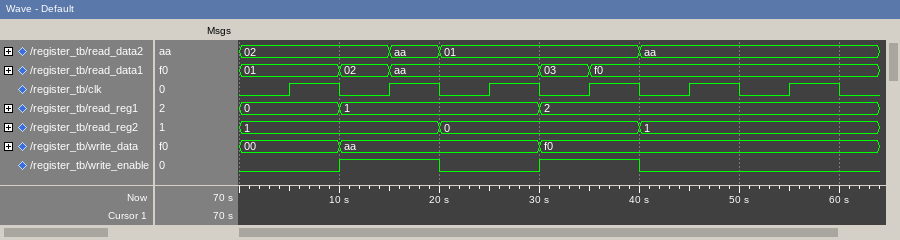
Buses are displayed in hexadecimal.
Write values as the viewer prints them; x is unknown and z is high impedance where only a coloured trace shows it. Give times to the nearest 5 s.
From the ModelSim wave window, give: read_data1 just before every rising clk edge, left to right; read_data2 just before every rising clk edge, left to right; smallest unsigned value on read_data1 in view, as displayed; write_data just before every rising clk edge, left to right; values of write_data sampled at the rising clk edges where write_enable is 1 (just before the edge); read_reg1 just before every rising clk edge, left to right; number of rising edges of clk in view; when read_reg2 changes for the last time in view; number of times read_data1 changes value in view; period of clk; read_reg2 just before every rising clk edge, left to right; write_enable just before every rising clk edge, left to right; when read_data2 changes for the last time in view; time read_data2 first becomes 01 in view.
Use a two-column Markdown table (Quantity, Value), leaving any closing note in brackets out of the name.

| Quantity | Value |
|---|---|
| read_data1 just before every rising clk edge, left to right | 01, 02, aa, 03, f0, f0 |
| read_data2 just before every rising clk edge, left to right | 02, 02, 01, 01, aa, aa |
| smallest unsigned value on read_data1 in view, as displayed | 01 |
| write_data just before every rising clk edge, left to right | 00, aa, aa, f0, f0, f0 |
| values of write_data sampled at the rising clk edges where write_enable is 1 | aa, f0 |
| read_reg1 just before every rising clk edge, left to right | 0, 1, 1, 2, 2, 2 |
| number of rising edges of clk in view | 6 |
| when read_reg2 changes for the last time in view | 40 s |
| number of times read_data1 changes value in view | 4 |
| period of clk | 10 s |
| read_reg2 just before every rising clk edge, left to right | 1, 1, 0, 0, 1, 1 |
| write_enable just before every rising clk edge, left to right | 0 1 0 1 0 0 |
| when read_data2 changes for the last time in view | 40 s |
| time read_data2 first becomes 01 in view | 20 s |
